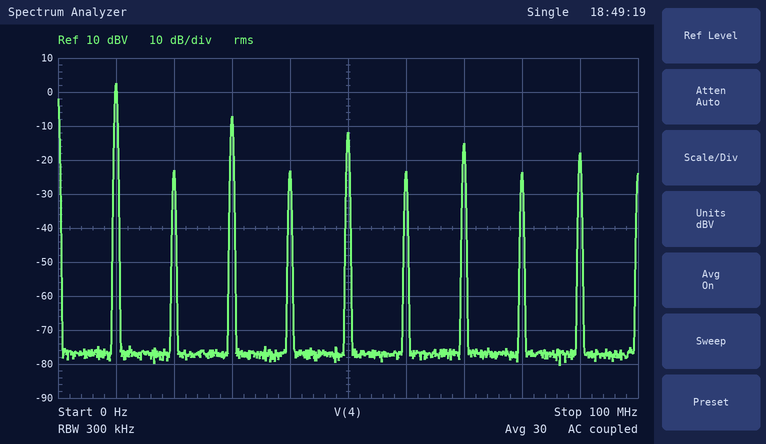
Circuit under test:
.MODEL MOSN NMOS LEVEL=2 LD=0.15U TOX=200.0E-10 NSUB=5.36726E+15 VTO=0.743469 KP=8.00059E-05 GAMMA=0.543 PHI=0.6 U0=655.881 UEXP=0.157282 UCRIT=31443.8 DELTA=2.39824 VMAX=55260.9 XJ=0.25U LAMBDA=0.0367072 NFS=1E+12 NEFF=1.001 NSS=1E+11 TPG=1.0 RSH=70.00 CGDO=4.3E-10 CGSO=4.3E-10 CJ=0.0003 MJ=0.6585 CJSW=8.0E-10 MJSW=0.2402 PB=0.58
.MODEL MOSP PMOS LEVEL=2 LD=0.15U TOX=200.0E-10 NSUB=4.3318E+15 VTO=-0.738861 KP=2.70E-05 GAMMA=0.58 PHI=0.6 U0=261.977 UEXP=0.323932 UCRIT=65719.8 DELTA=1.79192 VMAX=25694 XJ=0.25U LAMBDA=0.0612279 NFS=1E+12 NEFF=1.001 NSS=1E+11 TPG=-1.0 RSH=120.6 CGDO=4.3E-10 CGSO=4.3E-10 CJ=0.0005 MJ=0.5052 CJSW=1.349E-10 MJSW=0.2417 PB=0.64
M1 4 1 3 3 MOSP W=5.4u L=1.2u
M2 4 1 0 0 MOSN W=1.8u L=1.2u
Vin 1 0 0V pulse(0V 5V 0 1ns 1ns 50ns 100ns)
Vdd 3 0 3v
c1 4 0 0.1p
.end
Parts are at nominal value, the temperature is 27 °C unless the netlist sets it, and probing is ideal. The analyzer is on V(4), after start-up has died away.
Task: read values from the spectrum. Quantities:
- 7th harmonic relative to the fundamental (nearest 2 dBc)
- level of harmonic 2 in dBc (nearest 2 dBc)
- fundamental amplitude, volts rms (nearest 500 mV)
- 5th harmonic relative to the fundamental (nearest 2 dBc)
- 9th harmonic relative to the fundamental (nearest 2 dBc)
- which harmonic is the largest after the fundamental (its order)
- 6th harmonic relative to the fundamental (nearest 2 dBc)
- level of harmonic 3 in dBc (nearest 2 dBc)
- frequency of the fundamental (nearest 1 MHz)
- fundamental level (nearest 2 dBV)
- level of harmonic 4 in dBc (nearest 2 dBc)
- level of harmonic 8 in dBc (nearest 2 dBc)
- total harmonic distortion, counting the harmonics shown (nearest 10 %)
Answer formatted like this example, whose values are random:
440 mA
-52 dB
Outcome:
-18 dBc
-26 dBc
1.5 V
-14 dBc
-20 dBc
3
-26 dBc
-10 dBc
10 MHz
2 dBV
-26 dBc
-26 dBc
40 %
